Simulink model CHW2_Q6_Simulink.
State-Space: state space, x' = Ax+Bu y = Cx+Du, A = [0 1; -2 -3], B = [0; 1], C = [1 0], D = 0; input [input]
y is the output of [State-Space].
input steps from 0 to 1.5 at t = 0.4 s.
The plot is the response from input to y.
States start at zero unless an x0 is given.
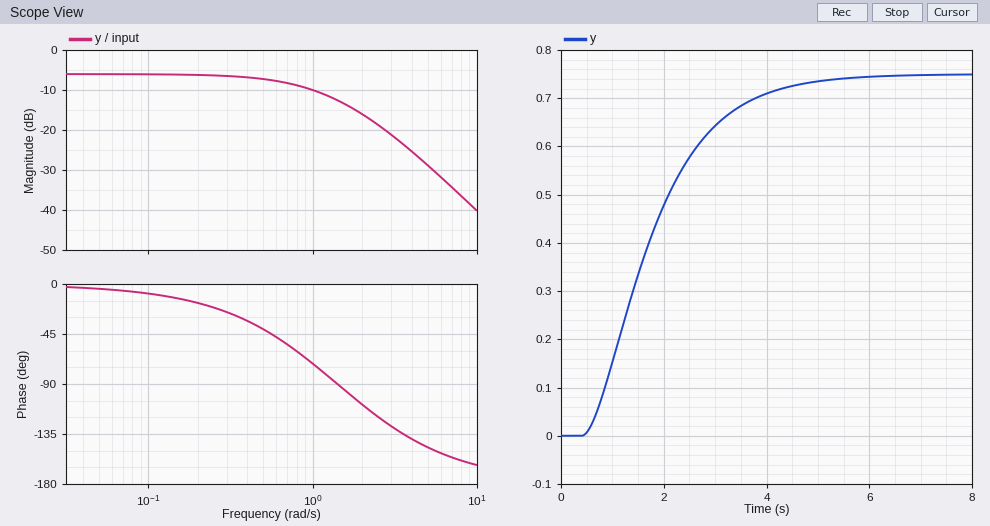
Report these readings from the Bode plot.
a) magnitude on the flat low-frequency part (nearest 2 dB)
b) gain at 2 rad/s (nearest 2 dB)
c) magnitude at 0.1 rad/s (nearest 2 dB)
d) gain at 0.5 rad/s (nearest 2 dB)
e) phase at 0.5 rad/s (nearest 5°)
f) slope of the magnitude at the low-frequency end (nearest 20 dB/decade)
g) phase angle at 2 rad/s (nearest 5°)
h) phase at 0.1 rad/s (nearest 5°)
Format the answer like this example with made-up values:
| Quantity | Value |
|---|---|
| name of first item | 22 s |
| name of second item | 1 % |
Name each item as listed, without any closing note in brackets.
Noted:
| Quantity | Value |
|---|---|
| magnitude on the flat low-frequency part | -6 dB |
| gain at 2 rad/s | -16 dB |
| magnitude at 0.1 rad/s | -6 dB |
| gain at 0.5 rad/s | -8 dB |
| phase at 0.5 rad/s | -40° |
| slope of the magnitude at the low-frequency end | 0 dB/decade |
| phase angle at 2 rad/s | -110° |
| phase at 0.1 rad/s | -10° |
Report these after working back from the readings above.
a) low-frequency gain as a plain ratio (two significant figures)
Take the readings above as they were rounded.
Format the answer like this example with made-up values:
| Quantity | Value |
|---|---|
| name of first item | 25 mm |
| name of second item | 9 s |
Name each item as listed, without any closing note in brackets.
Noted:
| Quantity | Value |
|---|---|
| low-frequency gain as a plain ratio | 0.50 |
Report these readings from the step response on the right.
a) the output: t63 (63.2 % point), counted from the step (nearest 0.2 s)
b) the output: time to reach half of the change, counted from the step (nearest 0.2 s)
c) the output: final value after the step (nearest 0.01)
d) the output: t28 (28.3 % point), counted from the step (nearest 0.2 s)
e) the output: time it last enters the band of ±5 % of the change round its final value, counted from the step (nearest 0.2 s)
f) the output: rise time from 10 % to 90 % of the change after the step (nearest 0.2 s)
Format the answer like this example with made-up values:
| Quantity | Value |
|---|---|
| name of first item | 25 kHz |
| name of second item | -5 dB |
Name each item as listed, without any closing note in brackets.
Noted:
| Quantity | Value |
|---|---|
| the output: t63 (63.2 % point), counted from the step | 1.6 s |
| the output: time to reach half of the change, counted from the step | 1.2 s |
| the output: final value after the step | 0.75 |
| the output: t28 (28.3 % point), counted from the step | 0.8 s |
| the output: time it last enters the band of ±5 % of the change round its final value, counted from the step | 3.6 s |
| the output: rise time from 10 % to 90 % of the change after the step | 2.6 s |
